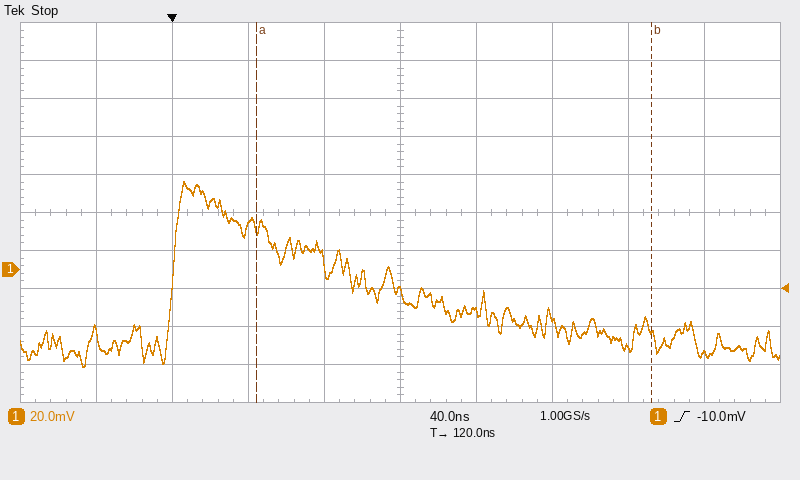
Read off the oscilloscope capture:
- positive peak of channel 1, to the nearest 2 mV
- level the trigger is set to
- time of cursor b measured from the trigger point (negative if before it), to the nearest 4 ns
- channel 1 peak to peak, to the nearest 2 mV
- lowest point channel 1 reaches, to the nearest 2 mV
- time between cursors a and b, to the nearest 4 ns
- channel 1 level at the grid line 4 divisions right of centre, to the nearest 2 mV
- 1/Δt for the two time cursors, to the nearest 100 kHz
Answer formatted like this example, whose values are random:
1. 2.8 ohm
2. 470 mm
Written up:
1. 46 mV
2. -10.0 mV
3. +252 ns
4. 98 mV
5. -52 mV
6. 208 ns
7. -44 mV
8. 4.8 MHz
